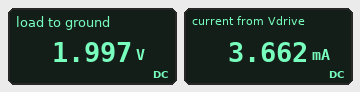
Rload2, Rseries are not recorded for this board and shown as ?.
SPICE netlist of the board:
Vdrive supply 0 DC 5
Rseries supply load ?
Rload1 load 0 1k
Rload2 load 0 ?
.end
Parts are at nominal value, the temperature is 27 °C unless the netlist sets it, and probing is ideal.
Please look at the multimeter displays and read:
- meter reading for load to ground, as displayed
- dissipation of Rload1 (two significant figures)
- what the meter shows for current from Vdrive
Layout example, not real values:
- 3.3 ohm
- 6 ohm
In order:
- 1.997 V
- 4.0 mW
- 3.662 mA
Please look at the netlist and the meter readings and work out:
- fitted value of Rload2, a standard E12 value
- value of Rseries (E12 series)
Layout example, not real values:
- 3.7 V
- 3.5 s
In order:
- 1.2 kΩ
- 820 Ω
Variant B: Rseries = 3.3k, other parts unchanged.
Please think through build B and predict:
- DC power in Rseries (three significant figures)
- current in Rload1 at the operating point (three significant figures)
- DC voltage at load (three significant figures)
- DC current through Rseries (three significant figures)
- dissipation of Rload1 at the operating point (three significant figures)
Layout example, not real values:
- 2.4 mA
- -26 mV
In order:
- 5.58 mW
- 709 µA
- 709 mV
- 1.30 mA
- 503 µW
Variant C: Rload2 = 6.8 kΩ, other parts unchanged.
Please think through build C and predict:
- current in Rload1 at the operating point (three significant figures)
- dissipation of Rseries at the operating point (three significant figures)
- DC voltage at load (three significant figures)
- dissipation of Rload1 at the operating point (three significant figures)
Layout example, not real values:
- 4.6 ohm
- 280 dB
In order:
- 2.58 mA
- 7.16 mW
- 2.58 V
- 6.64 mW
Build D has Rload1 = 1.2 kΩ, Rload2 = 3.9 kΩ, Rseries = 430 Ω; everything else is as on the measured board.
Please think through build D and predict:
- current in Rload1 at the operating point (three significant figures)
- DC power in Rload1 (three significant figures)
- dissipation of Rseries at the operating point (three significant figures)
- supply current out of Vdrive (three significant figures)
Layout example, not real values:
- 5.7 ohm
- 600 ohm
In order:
- 2.84 mA
- 9.66 mW
- 5.92 mW
- 3.71 mA
